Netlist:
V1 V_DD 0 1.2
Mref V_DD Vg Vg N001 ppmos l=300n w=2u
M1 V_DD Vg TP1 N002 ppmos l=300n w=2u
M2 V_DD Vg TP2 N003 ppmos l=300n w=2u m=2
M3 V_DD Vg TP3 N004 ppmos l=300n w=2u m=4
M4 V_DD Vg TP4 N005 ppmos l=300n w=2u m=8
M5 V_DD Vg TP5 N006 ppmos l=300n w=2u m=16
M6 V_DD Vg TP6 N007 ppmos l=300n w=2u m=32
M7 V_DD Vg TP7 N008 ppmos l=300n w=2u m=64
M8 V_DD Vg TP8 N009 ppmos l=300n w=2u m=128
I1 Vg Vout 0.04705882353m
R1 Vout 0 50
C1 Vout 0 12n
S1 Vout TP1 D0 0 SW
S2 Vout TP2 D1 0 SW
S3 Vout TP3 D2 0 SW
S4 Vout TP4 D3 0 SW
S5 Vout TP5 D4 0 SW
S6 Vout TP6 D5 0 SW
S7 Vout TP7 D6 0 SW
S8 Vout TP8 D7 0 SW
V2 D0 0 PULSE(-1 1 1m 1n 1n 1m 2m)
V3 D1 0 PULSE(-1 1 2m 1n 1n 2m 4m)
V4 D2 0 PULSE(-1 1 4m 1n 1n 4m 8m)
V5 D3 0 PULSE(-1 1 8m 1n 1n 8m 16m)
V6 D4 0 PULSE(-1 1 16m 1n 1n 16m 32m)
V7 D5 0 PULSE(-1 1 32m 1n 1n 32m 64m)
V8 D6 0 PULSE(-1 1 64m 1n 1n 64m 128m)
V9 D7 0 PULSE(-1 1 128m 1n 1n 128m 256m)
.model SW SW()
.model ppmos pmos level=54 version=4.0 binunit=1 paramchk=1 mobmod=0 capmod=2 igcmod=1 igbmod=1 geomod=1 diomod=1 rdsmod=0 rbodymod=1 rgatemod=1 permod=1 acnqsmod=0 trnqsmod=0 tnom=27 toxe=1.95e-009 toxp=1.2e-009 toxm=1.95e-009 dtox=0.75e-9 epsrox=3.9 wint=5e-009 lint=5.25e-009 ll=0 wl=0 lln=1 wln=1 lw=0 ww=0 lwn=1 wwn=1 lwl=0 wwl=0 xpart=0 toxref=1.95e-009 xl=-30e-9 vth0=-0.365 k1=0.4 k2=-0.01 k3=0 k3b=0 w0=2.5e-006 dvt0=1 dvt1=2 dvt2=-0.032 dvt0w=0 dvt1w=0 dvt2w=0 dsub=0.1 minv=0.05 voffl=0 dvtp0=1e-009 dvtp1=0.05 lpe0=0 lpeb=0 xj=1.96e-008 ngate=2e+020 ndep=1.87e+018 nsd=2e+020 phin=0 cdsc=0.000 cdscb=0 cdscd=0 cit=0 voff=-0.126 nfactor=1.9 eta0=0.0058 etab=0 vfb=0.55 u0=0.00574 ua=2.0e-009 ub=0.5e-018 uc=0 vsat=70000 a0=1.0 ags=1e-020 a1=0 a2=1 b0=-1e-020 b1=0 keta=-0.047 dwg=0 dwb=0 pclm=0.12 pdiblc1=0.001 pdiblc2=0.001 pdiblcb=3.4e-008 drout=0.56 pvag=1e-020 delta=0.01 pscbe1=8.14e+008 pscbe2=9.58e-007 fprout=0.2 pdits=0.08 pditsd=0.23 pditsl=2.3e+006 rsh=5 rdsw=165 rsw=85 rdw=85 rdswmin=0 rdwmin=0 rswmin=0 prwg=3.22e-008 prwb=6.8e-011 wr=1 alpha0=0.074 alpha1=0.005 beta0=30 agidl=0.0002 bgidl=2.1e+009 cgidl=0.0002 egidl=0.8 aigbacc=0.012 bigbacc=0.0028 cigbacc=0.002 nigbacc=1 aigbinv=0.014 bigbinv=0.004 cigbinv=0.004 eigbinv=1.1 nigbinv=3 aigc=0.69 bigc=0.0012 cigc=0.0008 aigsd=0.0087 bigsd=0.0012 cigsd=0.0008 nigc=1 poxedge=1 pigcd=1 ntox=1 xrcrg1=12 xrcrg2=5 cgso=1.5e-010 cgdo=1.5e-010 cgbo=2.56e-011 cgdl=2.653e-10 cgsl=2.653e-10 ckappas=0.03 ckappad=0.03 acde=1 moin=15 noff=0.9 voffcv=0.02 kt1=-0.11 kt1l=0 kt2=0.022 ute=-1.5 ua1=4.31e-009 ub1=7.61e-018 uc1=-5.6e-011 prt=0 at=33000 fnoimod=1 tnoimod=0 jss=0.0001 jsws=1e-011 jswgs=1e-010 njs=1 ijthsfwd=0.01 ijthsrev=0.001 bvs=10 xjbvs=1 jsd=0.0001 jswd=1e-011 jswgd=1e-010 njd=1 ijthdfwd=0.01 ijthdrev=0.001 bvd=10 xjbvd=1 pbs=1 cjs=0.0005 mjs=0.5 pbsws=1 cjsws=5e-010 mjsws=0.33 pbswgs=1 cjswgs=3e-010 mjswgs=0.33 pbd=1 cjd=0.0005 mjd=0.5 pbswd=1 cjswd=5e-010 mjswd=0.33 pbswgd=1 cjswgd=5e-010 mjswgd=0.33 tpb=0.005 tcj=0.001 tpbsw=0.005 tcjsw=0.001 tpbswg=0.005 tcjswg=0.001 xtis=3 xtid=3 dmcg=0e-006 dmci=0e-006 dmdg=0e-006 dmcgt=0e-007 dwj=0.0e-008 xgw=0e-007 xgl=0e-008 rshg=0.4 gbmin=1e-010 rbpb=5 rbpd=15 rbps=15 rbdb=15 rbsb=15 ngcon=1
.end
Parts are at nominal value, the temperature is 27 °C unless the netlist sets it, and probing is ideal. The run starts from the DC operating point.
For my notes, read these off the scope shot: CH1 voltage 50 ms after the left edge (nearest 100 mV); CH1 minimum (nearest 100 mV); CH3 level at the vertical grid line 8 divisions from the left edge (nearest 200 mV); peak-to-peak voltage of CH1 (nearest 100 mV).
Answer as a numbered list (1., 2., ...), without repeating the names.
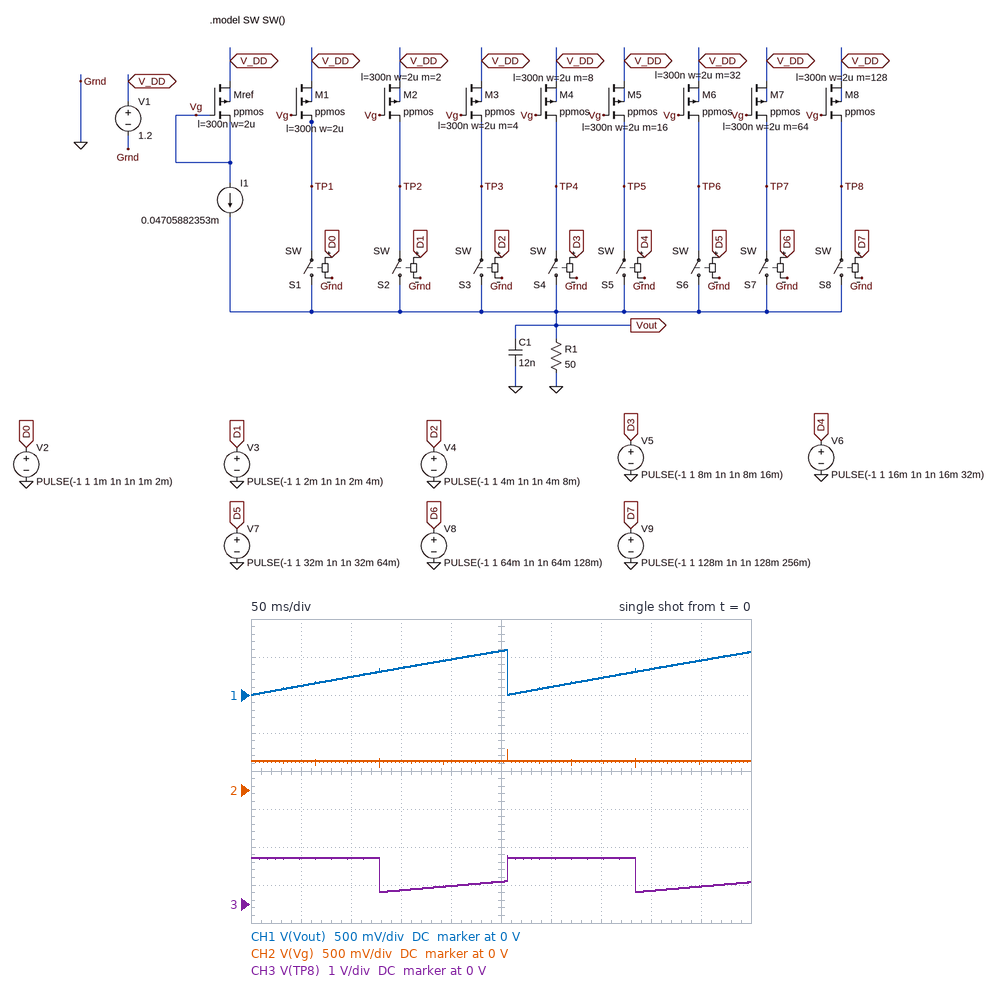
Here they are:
1. 100 mV
2. 0 V
3. 400 mV
4. 600 mV
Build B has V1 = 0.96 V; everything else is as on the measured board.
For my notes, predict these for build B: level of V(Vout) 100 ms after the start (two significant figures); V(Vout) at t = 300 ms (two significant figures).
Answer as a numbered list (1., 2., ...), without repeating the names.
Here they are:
1. 230 mV
2. 100 mV
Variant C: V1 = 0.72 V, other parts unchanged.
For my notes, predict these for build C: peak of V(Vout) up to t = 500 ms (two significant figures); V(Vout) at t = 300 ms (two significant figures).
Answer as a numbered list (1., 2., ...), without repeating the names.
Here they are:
1. 460 mV
2. 100 mV
